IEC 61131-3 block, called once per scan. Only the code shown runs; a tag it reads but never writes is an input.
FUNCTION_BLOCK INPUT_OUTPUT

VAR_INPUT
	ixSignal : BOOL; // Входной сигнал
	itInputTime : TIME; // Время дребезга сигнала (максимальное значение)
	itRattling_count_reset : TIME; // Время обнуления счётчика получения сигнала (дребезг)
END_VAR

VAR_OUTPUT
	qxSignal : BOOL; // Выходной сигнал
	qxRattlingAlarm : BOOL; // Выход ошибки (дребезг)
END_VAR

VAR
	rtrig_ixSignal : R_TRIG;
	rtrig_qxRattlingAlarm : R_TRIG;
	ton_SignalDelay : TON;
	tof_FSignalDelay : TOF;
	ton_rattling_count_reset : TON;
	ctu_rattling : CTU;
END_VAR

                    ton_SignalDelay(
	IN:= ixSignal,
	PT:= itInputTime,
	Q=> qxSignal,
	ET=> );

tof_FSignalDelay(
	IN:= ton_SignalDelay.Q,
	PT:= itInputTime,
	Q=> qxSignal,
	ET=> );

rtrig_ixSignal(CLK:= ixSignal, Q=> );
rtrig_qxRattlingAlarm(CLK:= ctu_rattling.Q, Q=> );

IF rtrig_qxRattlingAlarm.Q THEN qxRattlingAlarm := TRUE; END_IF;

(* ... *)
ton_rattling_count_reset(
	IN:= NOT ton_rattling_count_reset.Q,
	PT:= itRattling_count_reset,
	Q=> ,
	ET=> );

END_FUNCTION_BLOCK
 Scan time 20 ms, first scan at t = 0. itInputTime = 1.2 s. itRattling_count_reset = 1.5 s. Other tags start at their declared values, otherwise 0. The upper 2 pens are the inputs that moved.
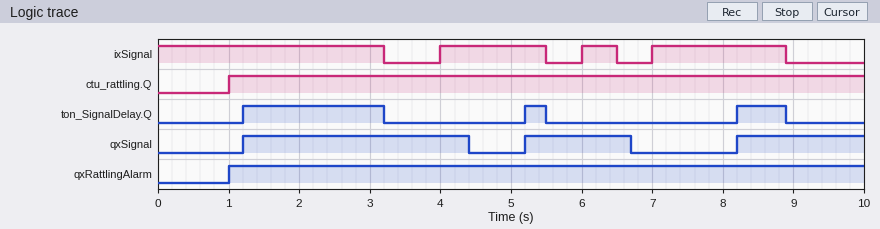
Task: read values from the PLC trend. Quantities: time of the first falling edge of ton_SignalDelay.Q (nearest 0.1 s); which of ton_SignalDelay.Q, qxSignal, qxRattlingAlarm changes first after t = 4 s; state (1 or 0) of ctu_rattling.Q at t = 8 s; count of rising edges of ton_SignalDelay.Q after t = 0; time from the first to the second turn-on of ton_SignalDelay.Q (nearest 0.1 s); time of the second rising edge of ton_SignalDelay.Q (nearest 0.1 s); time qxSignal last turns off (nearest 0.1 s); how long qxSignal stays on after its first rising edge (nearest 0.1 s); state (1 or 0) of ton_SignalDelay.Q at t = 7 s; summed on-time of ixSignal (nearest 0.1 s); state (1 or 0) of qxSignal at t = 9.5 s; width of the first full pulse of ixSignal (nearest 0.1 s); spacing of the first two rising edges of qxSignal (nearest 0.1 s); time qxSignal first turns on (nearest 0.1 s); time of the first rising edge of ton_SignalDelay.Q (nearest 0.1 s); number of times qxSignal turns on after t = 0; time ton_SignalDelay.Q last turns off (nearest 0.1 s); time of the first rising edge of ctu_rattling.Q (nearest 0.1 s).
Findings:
3.2 s
qxSignal
1
3
4.0 s
5.2 s
6.7 s
3.2 s
0
7.1 s
1
1.5 s
4.0 s
1.2 s
1.2 s
3
8.9 s
1.0 s
